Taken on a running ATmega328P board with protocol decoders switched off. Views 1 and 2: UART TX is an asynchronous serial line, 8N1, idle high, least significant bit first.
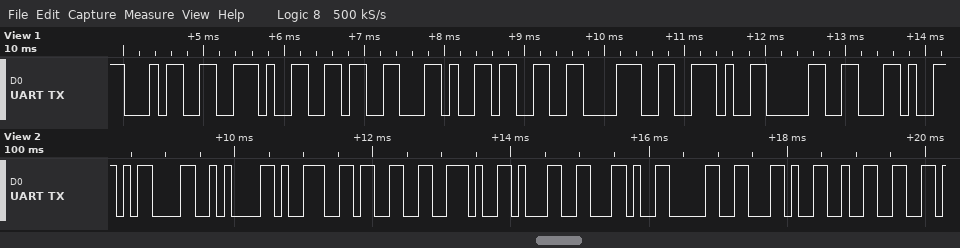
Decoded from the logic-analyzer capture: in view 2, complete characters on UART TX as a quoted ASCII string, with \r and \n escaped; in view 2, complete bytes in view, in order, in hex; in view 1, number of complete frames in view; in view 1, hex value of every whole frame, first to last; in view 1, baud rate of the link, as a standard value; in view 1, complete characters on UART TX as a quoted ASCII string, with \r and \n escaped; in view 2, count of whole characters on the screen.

"\r\n93.1,0,2"
0x0D 0x0A 0x39 0x33 0x2E 0x31 0x2C 0x30 0x2C 0x32
9
34 2E 36 2C 33 38 2E 30 2C
9600 baud
"4.6,38.0,"
10
